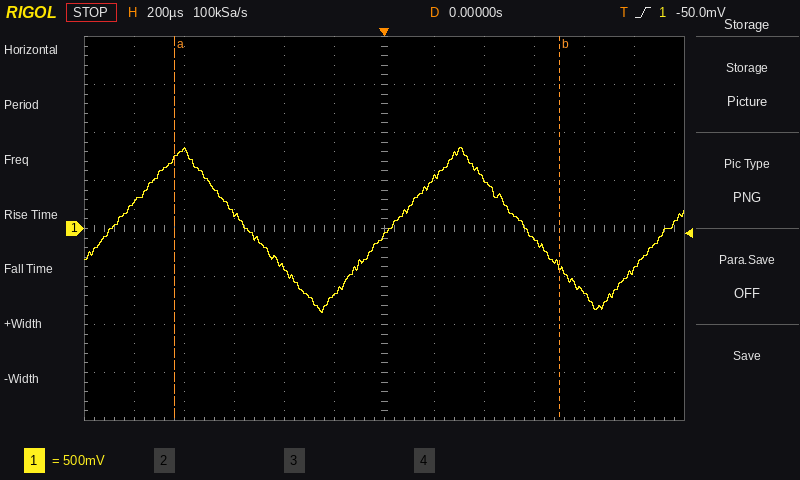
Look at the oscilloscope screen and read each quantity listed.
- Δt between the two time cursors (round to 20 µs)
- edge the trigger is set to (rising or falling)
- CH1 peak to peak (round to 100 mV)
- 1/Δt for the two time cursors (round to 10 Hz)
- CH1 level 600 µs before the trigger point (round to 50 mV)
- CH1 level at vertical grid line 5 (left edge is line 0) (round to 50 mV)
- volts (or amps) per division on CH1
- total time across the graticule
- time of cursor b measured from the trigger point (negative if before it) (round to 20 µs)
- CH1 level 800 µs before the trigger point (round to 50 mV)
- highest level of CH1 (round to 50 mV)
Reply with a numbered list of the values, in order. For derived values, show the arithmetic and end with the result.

1. 1.54 ms
2. rising
3. 1.70 V
4. 1 / 1.54 ms ≈ 650 Hz
5. 150 mV
6. -700 mV
7. 500 mV
8. 2.4 ms
9. +700 µs
10. 800 mV
11. 850 mV
